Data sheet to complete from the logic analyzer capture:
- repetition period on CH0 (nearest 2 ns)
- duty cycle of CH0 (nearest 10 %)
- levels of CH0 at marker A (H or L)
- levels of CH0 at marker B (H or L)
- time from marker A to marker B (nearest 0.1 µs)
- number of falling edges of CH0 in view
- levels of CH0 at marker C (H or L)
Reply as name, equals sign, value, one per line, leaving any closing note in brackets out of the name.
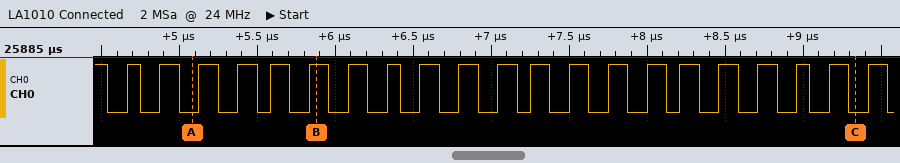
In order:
repetition period on CH0 = 238 ns
duty cycle of CH0 = 50 %
levels of CH0 at marker A = CH0=L
levels of CH0 at marker B = CH0=H
time from marker A to marker B = 0.8 µs
number of falling edges of CH0 in view = 22
levels of CH0 at marker C = CH0=L
